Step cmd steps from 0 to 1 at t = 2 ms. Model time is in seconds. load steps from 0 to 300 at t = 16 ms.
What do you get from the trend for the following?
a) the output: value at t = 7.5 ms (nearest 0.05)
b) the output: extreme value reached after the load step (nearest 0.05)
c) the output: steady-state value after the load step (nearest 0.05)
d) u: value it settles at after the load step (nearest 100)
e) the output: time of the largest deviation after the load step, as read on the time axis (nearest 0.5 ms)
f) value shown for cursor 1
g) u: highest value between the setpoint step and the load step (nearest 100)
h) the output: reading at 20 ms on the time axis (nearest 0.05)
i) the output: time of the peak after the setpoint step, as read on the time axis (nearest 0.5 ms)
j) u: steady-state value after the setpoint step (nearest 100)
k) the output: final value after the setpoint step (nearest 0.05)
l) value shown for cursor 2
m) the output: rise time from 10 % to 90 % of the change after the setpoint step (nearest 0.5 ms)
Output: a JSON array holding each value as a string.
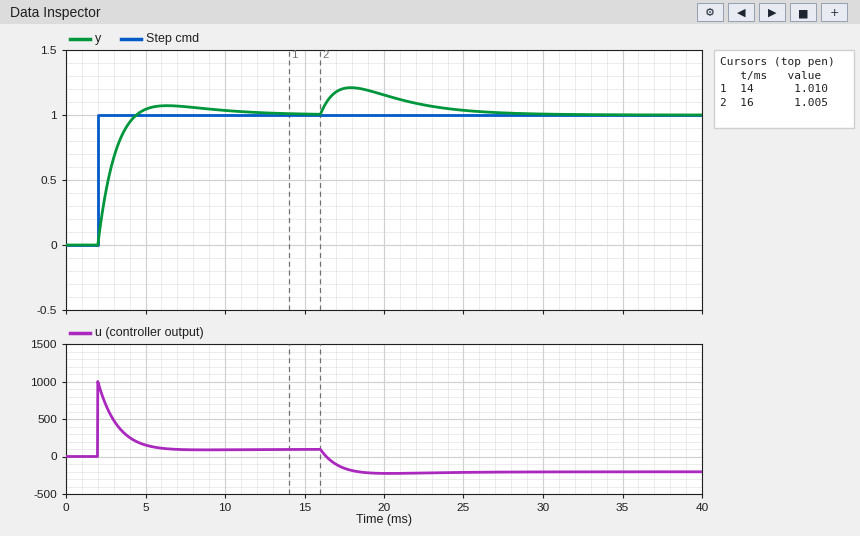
["1.05", "1.20", "1.00", "-200", "18.0 ms", "1.010", "1000", "1.15", "6.5 ms", "100", "1.00", "1.005", "1.5 ms"]
